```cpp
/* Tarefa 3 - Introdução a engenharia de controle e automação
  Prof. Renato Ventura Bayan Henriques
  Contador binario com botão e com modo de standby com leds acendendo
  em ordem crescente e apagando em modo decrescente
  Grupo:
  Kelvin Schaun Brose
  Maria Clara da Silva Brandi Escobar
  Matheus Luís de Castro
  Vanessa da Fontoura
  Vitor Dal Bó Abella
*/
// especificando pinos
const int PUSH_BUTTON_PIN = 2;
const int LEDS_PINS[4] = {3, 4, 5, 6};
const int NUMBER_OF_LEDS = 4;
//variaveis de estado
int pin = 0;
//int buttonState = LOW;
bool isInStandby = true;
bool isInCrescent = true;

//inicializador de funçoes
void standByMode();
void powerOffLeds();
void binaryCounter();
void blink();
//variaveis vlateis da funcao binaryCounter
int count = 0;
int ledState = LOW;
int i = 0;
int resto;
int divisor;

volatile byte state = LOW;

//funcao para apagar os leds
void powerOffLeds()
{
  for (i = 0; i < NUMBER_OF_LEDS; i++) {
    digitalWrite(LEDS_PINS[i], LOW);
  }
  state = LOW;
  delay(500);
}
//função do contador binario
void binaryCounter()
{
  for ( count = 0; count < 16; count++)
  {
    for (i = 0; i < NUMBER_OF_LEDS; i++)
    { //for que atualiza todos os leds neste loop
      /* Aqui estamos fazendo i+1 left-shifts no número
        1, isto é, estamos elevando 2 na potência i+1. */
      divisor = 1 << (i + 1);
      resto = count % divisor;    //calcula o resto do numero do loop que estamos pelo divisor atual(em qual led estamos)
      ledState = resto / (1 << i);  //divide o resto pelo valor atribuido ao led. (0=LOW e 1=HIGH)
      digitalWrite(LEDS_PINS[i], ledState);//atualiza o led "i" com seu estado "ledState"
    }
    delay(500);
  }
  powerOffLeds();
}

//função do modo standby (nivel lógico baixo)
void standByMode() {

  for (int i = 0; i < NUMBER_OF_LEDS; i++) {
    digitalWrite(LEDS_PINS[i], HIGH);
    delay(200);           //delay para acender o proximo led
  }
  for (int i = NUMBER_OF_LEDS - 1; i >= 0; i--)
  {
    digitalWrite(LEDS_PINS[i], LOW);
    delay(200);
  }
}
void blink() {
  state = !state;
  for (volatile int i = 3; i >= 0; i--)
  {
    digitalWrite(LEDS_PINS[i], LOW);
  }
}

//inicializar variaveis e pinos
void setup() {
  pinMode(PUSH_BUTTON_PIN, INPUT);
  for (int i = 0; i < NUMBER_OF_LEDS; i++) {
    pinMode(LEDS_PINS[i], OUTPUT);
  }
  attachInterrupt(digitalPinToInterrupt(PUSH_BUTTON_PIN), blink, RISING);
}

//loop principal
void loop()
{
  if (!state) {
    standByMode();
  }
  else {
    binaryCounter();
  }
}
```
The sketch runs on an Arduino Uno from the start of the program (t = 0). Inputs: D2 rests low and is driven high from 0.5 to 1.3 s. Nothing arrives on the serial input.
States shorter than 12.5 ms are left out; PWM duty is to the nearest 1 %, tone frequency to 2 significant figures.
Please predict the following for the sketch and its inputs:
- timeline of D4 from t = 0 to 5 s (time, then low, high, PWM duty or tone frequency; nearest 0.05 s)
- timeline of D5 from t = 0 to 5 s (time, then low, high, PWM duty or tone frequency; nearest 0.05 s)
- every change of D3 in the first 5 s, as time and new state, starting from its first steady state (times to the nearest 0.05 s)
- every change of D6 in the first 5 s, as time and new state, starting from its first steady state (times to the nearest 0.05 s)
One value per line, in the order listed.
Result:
0 s low; 0.2 s high; 0.5 s low; 2.6 s high; 3.6 s low; 4.6 s high
0 s low; 0.4 s high; 0.5 s low; 3.6 s high
0 s high; 0.5 s low; 2.1 s high; 2.6 s low; 3.1 s high; 3.6 s low; 4.1 s high; 4.6 s low
0 s low; 0.6 s high; 0.8 s low
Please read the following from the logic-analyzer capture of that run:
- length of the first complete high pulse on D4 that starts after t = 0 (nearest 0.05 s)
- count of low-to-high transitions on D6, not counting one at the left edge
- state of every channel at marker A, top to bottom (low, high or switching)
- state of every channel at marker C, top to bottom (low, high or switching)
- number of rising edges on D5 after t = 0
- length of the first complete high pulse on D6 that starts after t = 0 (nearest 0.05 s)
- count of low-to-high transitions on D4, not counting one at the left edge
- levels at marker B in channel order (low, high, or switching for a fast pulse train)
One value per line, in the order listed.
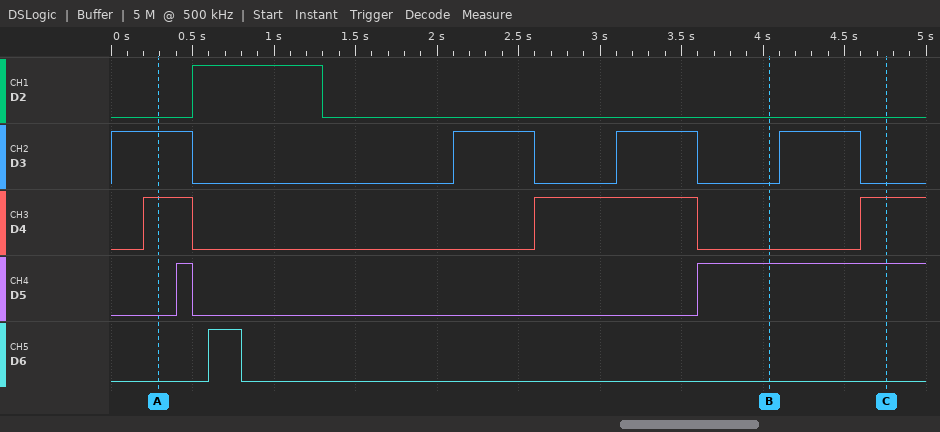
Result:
0.30 s
1
D2 low, D3 high, D4 high, D5 low, D6 low
D2 low, D3 low, D4 high, D5 high, D6 low
2
0.20 s
3
D2 low, D3 low, D4 low, D5 high, D6 low
